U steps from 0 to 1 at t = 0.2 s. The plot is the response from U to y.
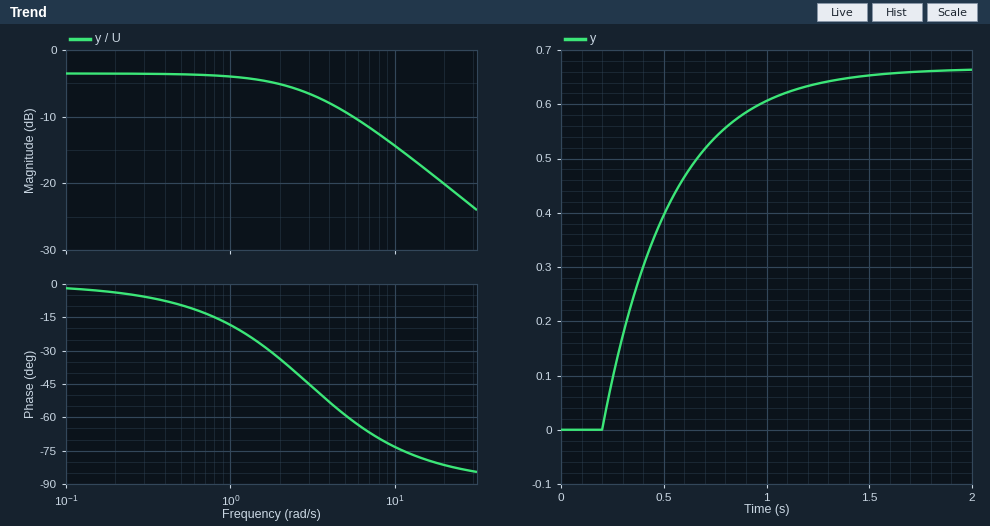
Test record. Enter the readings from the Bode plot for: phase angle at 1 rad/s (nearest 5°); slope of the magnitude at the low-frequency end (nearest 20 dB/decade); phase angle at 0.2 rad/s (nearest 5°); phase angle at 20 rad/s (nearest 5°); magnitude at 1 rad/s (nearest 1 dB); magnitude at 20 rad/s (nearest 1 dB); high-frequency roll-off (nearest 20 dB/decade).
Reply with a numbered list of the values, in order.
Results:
1. -20°
2. 0 dB/decade
3. -5°
4. -80°
5. -4 dB
6. -20 dB
7. -20 dB/decade
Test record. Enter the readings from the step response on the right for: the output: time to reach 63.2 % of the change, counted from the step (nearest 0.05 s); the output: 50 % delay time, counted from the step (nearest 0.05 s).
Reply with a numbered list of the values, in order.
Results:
1. 0.35 s
2. 0.25 s
